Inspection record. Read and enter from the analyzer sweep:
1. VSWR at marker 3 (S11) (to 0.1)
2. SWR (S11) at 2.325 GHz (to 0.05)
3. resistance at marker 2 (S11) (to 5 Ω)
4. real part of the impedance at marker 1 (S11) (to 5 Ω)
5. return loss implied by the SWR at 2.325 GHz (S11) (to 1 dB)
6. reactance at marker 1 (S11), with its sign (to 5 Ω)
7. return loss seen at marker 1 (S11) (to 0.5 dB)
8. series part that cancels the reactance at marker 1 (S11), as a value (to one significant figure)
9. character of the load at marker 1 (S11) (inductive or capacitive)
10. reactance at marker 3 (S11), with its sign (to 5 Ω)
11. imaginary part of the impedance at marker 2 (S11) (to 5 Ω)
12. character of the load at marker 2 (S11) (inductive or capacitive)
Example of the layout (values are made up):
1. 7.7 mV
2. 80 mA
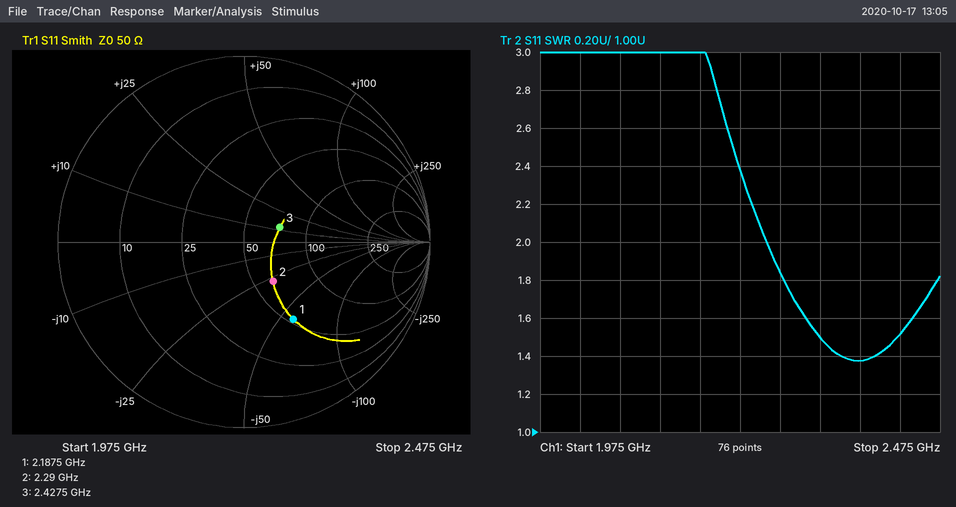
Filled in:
1. 1.5
2. 1.50
3. 60 Ω
4. 55 Ω
5. 14 dB
6. -60 Ω
7. 6.0 dB
8. 4 nH
9. capacitive
10. +10 Ω
11. -30 Ω
12. capacitive
